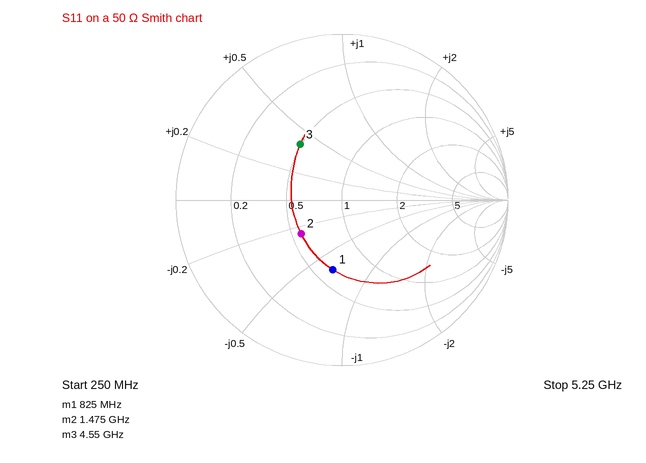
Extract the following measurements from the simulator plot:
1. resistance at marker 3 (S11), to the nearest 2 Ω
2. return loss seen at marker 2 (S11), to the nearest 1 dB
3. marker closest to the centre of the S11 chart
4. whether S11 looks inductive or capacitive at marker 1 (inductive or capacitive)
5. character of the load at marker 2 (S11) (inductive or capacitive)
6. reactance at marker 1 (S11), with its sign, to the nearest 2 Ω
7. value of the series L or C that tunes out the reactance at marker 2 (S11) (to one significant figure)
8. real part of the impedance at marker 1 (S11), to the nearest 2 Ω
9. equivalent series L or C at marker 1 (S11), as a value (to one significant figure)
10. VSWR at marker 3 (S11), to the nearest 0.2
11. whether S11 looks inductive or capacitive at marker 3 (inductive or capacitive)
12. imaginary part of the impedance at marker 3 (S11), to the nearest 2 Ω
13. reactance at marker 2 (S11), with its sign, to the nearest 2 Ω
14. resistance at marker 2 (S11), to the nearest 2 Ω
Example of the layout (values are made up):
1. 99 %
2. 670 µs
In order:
1. 24 Ω
2. 10 dB
3. marker 2
4. capacitive
5. capacitive
6. -32 Ω
7. 1 nH
8. 32 Ω
9. 6 pF
10. 2.4
11. inductive
12. +20 Ω
13. -12 Ω
14. 28 Ω
